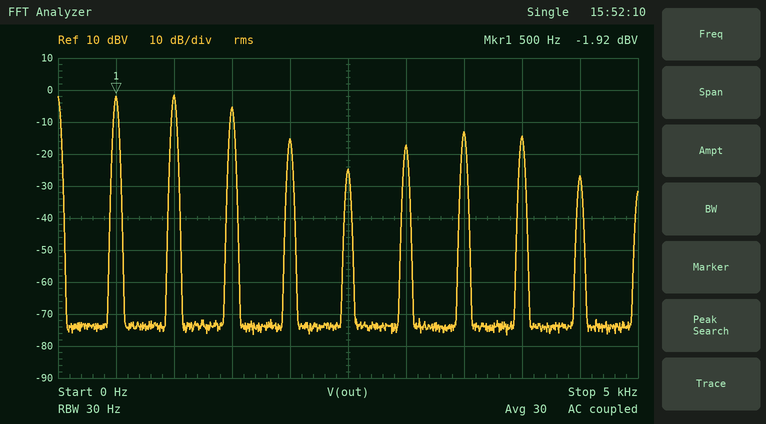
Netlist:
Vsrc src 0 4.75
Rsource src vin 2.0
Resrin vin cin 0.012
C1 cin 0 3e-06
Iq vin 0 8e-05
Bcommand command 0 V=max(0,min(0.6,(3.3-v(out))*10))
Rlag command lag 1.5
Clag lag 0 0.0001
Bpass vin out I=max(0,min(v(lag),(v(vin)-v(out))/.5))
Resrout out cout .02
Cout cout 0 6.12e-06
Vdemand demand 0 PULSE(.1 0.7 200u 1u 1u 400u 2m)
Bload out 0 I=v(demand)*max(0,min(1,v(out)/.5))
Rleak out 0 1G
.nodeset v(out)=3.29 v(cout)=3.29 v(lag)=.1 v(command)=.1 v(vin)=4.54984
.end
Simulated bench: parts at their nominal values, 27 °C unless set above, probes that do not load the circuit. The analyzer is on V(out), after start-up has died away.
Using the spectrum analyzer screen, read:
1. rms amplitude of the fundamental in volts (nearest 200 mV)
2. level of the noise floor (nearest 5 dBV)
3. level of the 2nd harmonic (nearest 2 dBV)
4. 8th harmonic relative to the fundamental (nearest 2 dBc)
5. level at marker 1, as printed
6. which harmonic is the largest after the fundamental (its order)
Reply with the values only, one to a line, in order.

800 mV
-75 dBV
-2 dBV
-12 dBc
-1.92 dBV
2
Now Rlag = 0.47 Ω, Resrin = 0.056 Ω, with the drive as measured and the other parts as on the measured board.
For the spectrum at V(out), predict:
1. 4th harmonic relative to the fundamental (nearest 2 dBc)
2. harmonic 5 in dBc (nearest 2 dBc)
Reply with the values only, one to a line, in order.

-8 dBc
-18 dBc
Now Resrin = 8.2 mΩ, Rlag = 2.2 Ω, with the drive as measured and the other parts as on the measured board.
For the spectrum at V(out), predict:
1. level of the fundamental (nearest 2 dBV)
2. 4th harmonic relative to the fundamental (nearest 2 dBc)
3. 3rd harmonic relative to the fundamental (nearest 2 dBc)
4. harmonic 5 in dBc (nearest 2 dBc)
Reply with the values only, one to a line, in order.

0 dBV
-16 dBc
-6 dBc
-30 dBc
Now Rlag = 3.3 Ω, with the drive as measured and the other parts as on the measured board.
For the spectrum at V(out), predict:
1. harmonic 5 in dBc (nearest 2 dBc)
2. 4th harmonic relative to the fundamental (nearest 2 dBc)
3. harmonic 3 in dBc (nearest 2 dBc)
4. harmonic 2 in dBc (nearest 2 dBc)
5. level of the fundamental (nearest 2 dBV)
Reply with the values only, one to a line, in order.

-18 dBc
-12 dBc
-8 dBc
-2 dBc
0 dBV
